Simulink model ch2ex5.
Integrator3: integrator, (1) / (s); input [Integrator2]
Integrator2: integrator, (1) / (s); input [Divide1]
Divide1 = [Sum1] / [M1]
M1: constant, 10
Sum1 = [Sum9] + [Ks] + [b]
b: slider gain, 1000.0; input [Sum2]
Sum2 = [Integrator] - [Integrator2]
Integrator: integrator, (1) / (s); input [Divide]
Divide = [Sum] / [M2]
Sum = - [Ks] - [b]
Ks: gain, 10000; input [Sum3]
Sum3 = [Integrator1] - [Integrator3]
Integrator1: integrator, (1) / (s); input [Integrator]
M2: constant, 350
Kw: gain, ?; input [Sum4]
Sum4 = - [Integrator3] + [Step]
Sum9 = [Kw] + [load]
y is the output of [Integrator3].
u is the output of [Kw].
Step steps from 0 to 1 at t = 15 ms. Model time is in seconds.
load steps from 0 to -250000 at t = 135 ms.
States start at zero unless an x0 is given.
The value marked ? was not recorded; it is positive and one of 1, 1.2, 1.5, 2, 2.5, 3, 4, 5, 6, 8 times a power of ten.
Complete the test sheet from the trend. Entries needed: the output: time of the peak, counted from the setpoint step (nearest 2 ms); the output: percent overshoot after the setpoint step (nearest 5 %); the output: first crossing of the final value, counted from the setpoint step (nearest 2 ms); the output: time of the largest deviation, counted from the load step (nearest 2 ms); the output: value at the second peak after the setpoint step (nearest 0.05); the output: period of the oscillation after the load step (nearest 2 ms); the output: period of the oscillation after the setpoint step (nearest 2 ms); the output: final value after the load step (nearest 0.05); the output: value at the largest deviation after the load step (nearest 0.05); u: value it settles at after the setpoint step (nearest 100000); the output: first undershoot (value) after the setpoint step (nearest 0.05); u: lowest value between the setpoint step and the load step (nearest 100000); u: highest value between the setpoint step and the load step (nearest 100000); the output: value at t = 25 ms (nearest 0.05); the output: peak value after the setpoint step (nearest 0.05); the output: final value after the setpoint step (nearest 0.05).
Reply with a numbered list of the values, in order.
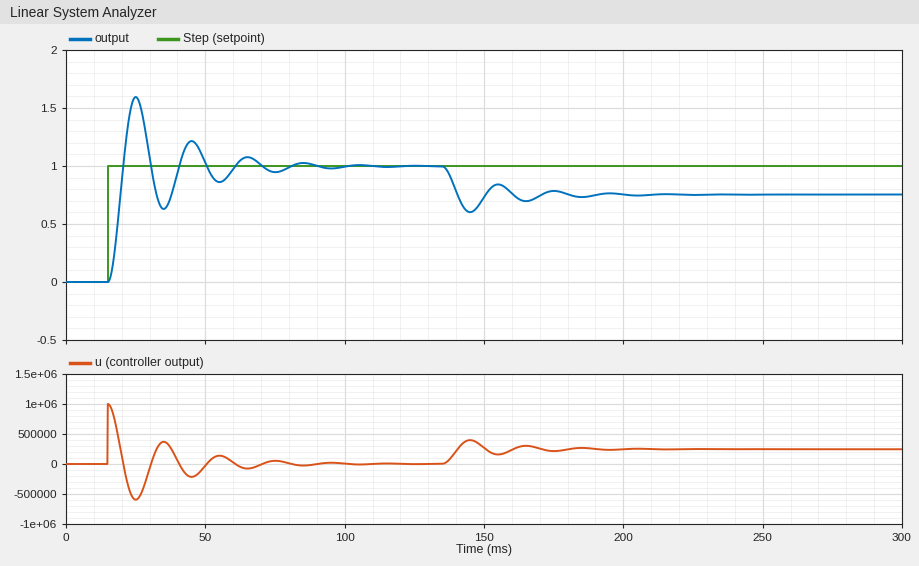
1. 10 ms
2. 60 %
3. 6 ms
4. 10 ms
5. 1.20
6. 20 ms
7. 20 ms
8. 0.75
9. 0.60
10. 0
11. 0.65
12. -600000
13. 1000000
14. 1.60
15. 1.60
16. 1.00
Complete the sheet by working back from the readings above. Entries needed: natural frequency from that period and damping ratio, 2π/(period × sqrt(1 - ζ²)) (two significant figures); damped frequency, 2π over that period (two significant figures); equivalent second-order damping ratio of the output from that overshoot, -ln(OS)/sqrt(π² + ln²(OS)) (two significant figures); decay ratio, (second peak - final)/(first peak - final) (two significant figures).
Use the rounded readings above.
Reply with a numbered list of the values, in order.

1. 0.32 rad/ms
2. 0.31 rad/ms
3. 0.16
4. 0.33
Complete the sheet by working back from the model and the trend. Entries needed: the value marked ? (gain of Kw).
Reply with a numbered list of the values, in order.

1. 1e+06
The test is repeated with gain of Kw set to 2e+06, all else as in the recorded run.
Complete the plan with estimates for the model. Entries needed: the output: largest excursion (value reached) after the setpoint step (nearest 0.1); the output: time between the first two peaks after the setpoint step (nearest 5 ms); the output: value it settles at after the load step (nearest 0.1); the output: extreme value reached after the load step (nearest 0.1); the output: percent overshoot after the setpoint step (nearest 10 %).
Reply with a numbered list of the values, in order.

1. 1.7
2. 15 ms
3. 0.9
4. 0.8
5. 70 %
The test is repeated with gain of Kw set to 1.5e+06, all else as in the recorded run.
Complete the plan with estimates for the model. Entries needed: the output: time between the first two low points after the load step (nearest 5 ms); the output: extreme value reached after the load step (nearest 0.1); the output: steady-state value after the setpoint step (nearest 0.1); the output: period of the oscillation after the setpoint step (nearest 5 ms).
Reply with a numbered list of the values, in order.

1. 15 ms
2. 0.7
3. 1.0
4. 15 ms
